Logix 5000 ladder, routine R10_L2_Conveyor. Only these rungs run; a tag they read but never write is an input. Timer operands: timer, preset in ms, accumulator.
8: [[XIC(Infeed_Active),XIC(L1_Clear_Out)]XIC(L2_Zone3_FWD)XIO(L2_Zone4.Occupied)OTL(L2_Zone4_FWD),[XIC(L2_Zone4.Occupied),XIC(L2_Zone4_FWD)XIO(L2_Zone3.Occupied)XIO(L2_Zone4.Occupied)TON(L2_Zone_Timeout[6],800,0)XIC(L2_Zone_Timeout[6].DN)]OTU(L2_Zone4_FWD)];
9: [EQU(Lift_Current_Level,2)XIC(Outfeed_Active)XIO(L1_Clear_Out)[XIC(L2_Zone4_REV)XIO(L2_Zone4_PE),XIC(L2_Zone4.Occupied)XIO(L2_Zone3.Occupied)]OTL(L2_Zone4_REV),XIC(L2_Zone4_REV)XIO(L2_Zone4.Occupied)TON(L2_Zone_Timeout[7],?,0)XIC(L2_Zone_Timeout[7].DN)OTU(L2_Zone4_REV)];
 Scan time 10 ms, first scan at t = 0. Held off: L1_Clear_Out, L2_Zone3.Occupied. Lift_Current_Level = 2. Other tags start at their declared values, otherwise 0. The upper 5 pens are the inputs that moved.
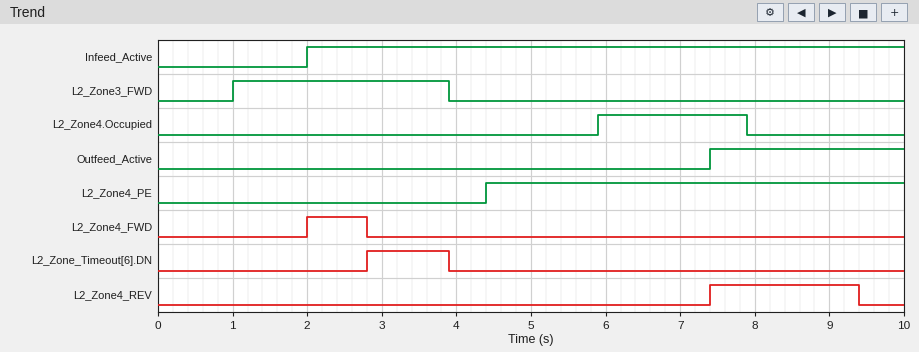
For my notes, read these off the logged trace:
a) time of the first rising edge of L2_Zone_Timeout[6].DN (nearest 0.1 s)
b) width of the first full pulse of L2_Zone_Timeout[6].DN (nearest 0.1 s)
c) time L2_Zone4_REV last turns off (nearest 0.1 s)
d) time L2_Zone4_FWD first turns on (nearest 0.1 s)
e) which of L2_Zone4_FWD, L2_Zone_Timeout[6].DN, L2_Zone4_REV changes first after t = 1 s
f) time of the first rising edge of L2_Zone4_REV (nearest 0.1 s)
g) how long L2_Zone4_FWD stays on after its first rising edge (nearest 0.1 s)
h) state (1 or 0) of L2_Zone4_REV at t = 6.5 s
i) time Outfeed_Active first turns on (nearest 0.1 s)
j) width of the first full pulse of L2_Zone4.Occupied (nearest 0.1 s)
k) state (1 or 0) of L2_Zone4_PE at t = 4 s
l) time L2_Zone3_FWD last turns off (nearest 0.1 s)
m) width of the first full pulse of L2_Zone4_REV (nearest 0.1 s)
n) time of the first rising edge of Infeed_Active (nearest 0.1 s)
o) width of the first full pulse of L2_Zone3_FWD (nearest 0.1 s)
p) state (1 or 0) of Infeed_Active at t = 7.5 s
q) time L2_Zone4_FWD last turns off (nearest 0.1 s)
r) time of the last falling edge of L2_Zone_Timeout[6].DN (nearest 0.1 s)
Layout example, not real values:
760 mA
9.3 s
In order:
2.8 s
1.1 s
9.4 s
2.0 s
L2_Zone4_FWD
7.4 s
0.8 s
0
7.4 s
2.0 s
0
3.9 s
2.0 s
2.0 s
2.9 s
1
2.8 s
3.9 s
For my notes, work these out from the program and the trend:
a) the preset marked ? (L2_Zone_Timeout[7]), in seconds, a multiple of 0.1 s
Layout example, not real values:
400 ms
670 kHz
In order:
1.5 s
